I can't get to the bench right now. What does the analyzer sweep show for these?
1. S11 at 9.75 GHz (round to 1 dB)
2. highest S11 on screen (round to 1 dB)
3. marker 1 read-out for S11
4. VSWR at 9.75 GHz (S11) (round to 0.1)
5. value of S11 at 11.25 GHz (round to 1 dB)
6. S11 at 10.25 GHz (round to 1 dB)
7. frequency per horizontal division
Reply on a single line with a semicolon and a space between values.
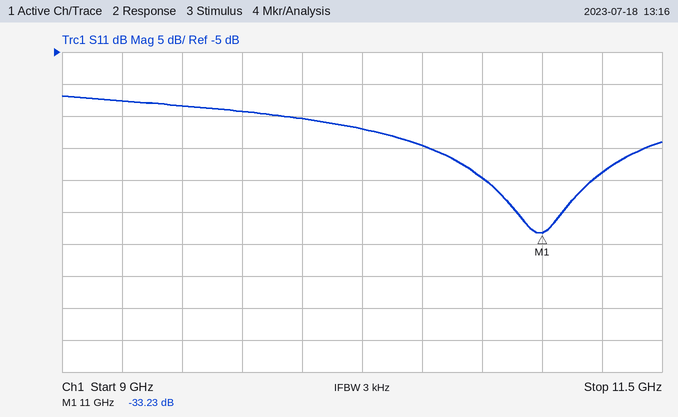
-14 dB; -12 dB; -33.23 dB; 1.5; -24 dB; -17 dB; 250 MHz
